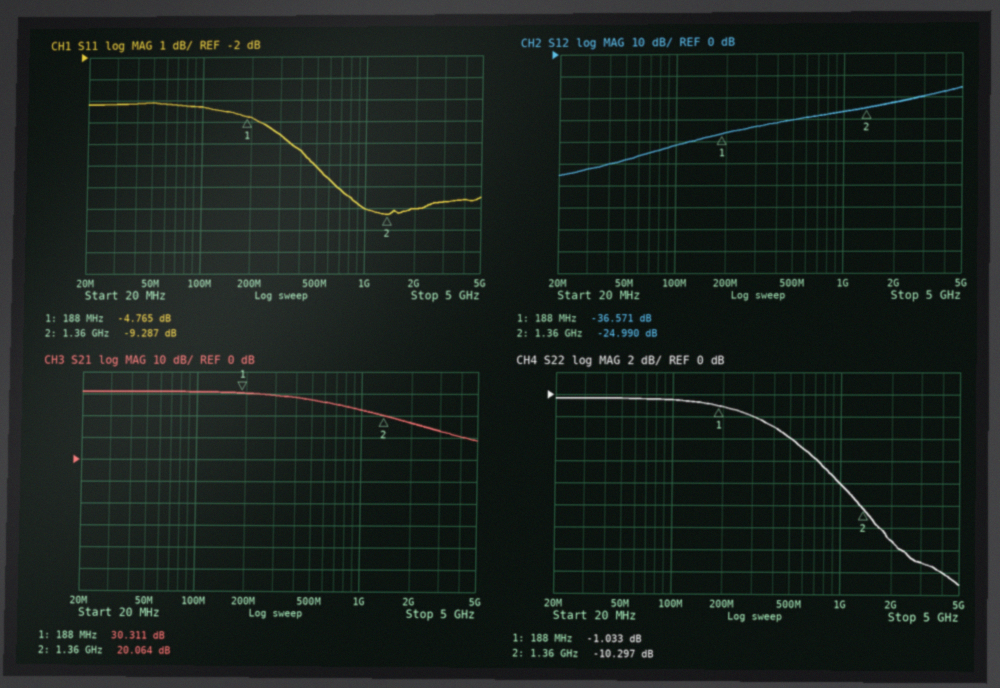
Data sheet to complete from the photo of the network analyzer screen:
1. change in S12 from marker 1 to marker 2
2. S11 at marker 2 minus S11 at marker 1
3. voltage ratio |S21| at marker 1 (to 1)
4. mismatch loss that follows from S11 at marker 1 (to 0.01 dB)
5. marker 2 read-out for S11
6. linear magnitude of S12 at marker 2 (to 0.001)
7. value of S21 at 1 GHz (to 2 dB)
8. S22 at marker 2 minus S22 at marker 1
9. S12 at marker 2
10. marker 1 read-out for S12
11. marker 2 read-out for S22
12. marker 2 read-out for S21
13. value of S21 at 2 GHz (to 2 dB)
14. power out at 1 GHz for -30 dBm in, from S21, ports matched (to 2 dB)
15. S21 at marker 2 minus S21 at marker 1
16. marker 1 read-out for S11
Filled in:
11.581 dB
-4.522 dB
33
1.76 dB
-9.287 dB
0.056
22 dB
-9.264 dB
-24.990 dB
-36.571 dB
-10.297 dB
20.064 dB
16 dB
-8 dBm
-10.247 dB
-4.765 dB
